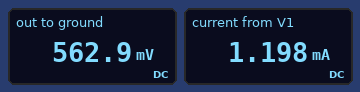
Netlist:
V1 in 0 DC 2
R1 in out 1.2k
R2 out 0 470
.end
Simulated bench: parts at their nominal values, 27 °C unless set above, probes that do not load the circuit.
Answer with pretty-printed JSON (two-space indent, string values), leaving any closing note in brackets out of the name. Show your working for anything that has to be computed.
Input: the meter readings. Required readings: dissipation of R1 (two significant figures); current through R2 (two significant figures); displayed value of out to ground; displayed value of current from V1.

{
  "dissipation of R1": "(2 V - 562.9 mV)^2 / 1.2 kΩ = 1.7 mW",
  "current through R2": "(562.9 mV) / 470 Ω = 1.2 mA",
  "displayed value of out to ground": "562.9 mV",
  "displayed value of current from V1": "1.198 mA"
}
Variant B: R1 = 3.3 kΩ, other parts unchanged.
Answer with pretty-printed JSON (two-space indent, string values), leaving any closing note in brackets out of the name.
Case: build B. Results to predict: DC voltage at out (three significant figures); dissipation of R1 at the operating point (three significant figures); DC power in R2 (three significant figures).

{
  "DC voltage at out": "249 mV",
  "dissipation of R1 at the operating point": "929 µW",
  "DC power in R2": "132 µW"
}
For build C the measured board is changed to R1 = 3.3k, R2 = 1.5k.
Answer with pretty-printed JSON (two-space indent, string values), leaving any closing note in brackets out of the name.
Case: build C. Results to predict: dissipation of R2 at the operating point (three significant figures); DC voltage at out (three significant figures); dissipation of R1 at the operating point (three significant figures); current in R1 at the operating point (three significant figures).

{
  "dissipation of R2 at the operating point": "260 µW",
  "DC voltage at out": "625 mV",
  "dissipation of R1 at the operating point": "573 µW",
  "current in R1 at the operating point": "417 µA"
}
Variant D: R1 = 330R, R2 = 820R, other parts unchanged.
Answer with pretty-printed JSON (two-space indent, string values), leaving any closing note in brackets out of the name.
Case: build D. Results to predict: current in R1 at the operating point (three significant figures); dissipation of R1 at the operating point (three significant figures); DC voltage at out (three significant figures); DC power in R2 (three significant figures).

{
  "current in R1 at the operating point": "1.74 mA",
  "dissipation of R1 at the operating point": "998 µW",
  "DC voltage at out": "1.43 V",
  "DC power in R2": "2.48 mW"
}
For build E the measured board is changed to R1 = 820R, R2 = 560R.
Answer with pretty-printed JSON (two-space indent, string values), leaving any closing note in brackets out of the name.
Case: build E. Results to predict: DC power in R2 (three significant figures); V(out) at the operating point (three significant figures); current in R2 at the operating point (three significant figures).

{
  "DC power in R2": "1.18 mW",
  "V(out) at the operating point": "812 mV",
  "current in R2 at the operating point": "1.45 mA"
}
